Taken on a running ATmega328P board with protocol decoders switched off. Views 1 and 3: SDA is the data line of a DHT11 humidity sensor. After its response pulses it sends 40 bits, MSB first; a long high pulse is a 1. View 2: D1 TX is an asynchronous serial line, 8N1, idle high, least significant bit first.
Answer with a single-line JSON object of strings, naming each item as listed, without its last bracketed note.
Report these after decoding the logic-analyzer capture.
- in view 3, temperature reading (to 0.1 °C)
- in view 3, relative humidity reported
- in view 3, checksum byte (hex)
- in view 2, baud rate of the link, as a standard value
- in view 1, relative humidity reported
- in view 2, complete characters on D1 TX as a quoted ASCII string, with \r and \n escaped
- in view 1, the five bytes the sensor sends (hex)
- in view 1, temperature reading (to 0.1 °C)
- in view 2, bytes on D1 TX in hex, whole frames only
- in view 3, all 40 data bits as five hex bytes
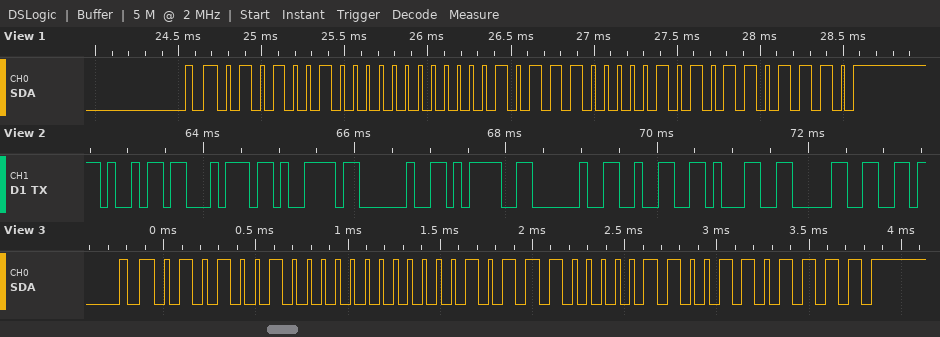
{"in view 3, temperature reading": "23.6 °C", "in view 3, relative humidity reported": "82 %", "in view 3, checksum byte": "0x6F", "in view 2, baud rate of the link, as a standard value": "9600 baud", "in view 1, relative humidity reported": "82 %", "in view 2, complete characters on D1 TX as a quoted ASCII string, with \\r and \\n escaped": "\"ity = 210\"", "in view 1, the five bytes the sensor sends": "52 00 17 05 6E", "in view 1, temperature reading": "23.5 °C", "in view 2, bytes on D1 TX in hex, whole frames only": "0x69 0x74 0x79 0x20 0x3D 0x20 0x32 0x31 0x30", "in view 3, all 40 data bits as five hex bytes": "52 00 17 06 6F"}
